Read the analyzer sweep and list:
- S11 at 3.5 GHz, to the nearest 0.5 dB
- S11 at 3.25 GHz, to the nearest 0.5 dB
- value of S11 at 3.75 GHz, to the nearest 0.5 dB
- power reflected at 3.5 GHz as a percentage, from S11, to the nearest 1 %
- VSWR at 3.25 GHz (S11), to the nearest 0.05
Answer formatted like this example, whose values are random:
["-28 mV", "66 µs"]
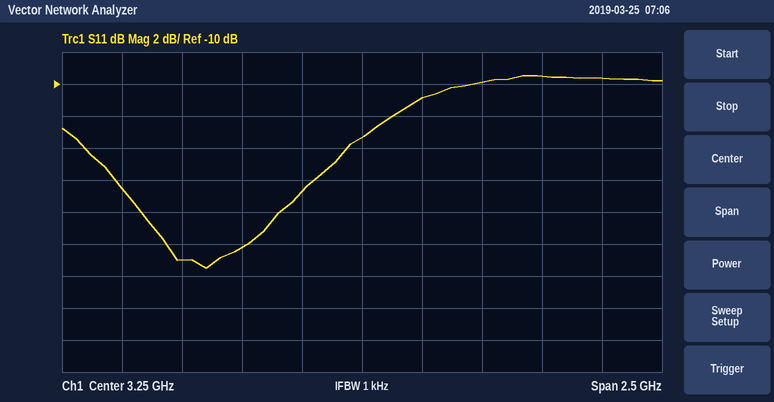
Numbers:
["-11.0 dB", "-13.5 dB", "-10.0 dB", "8 %", "1.55"]
